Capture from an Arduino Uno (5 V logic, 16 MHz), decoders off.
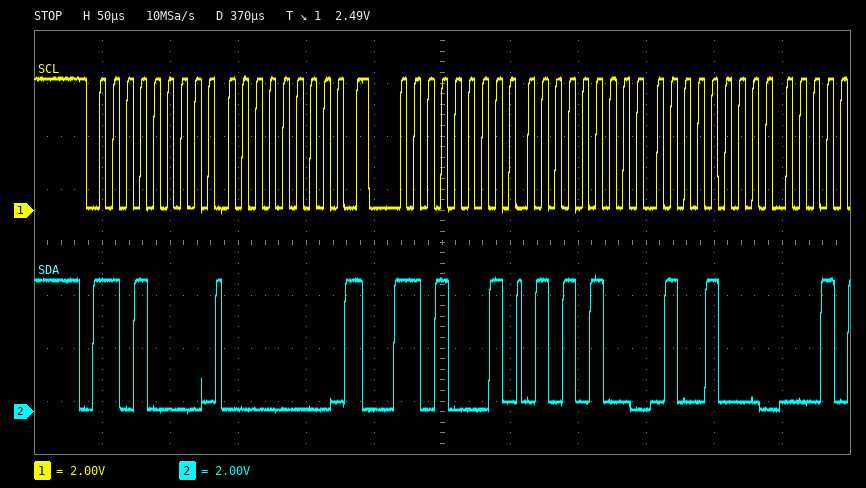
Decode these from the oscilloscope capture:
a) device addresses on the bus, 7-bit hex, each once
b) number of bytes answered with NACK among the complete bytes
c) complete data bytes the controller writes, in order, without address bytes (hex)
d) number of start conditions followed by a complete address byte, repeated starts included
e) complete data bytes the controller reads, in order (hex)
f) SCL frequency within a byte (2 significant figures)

0x68
0
00
2
54 48
100 kHz
